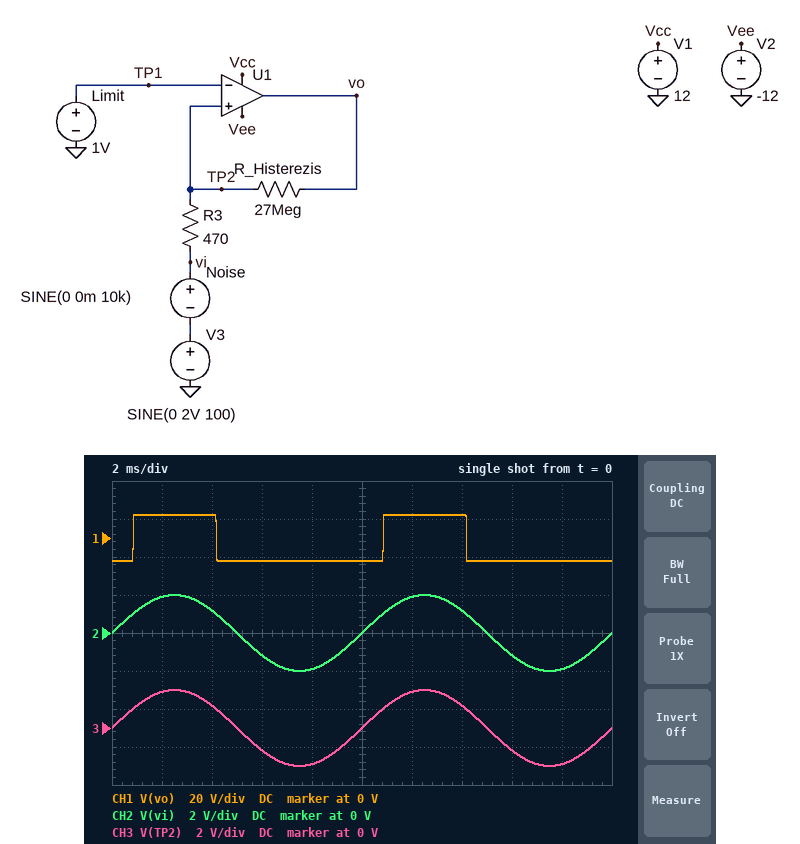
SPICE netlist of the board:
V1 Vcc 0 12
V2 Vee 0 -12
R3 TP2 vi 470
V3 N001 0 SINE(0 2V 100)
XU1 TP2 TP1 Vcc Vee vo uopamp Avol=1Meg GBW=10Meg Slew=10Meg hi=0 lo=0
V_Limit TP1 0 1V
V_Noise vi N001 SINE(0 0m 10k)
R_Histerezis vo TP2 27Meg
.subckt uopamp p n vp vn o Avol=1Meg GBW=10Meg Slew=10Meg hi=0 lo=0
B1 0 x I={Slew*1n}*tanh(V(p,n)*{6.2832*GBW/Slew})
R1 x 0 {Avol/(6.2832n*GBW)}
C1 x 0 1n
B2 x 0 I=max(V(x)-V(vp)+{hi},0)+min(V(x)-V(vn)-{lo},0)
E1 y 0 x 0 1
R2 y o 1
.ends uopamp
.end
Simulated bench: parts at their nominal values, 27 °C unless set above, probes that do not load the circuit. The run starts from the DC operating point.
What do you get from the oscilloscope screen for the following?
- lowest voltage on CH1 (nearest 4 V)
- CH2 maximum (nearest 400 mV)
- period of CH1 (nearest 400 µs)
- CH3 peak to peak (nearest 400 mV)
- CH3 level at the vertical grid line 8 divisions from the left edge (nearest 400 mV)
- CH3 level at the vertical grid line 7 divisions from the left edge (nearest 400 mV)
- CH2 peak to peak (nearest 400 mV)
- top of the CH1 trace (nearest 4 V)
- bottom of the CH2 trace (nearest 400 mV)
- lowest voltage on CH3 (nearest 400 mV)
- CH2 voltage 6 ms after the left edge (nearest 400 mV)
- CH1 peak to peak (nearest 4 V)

-12 V
2.0 V
10.0 ms
4.0 V
-1.2 V
1.2 V
4.0 V
12 V
-2.0 V
-2.0 V
-1.2 V
24 V
